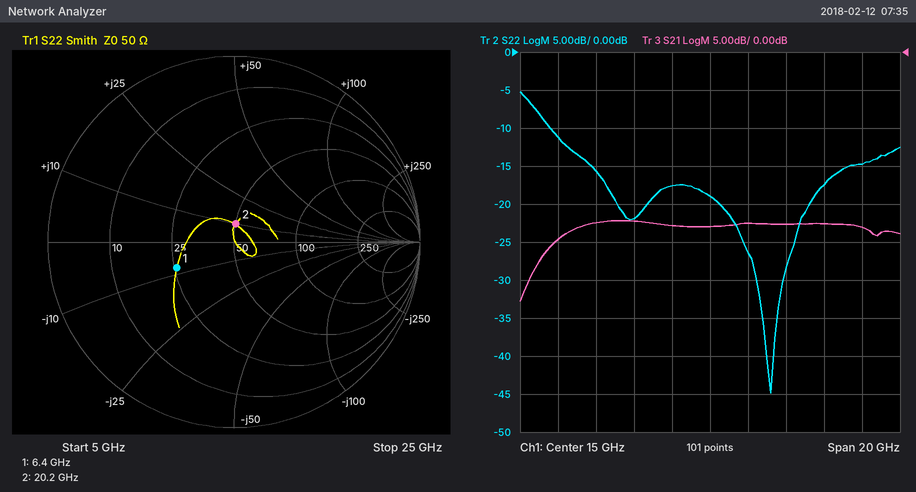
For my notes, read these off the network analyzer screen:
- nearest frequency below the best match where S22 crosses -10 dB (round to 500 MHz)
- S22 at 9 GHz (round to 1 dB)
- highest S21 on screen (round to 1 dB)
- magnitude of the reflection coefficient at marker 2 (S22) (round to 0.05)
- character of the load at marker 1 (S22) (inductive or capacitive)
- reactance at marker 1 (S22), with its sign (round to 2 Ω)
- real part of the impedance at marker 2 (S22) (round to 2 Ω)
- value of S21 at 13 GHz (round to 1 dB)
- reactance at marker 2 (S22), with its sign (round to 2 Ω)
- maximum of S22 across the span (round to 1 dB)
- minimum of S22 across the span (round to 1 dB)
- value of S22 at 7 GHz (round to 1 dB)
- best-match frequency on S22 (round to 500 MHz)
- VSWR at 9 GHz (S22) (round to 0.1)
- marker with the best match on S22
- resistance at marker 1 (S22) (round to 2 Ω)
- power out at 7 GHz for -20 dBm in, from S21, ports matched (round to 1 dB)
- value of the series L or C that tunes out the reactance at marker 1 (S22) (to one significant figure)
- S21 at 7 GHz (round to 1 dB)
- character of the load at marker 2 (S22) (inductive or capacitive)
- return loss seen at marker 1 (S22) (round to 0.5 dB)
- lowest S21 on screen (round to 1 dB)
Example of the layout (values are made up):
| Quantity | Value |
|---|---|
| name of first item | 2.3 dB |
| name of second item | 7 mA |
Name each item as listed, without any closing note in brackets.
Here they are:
| Quantity | Value |
|---|---|
| nearest frequency below the best match where S22 crosses -10 dB | 6.5 GHz |
| S22 at 9 GHz | -16 dB |
| highest S21 on screen | -22 dB |
| magnitude of the reflection coefficient at marker 2 (S22) | 0.10 |
| character of the load at marker 1 (S22) | capacitive |
| reactance at marker 1 (S22), with its sign | -8 Ω |
| real part of the impedance at marker 2 (S22) | 50 Ω |
| value of S21 at 13 GHz | -23 dB |
| reactance at marker 2 (S22), with its sign | +10 Ω |
| maximum of S22 across the span | -5 dB |
| minimum of S22 across the span | -45 dB |
| value of S22 at 7 GHz | -11 dB |
| best-match frequency on S22 | 18.0 GHz |
| VSWR at 9 GHz (S22) | 1.4 |
| marker with the best match on S22 | marker 2 |
| resistance at marker 1 (S22) | 26 Ω |
| power out at 7 GHz for -20 dBm in, from S21, ports matched | -45 dBm |
| value of the series L or C that tunes out the reactance at marker 1 (S22) | 200 pH |
| S21 at 7 GHz | -25 dB |
| character of the load at marker 2 (S22) | inductive |
| return loss seen at marker 1 (S22) | 9.5 dB |
| lowest S21 on screen | -33 dB |
